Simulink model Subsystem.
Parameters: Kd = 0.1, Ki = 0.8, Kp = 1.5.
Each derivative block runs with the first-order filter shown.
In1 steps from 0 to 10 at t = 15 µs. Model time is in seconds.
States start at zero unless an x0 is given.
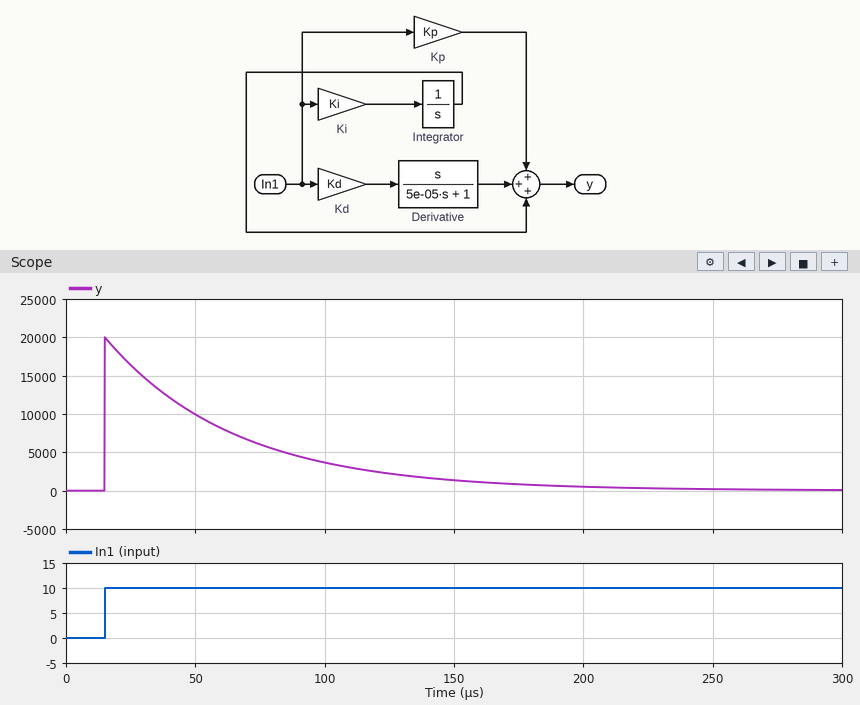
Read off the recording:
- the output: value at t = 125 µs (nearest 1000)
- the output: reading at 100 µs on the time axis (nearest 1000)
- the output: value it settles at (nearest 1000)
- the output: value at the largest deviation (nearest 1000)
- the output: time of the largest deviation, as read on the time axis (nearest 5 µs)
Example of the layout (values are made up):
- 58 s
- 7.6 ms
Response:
- 2000
- 4000
- 0
- 20000
- 15 µs
